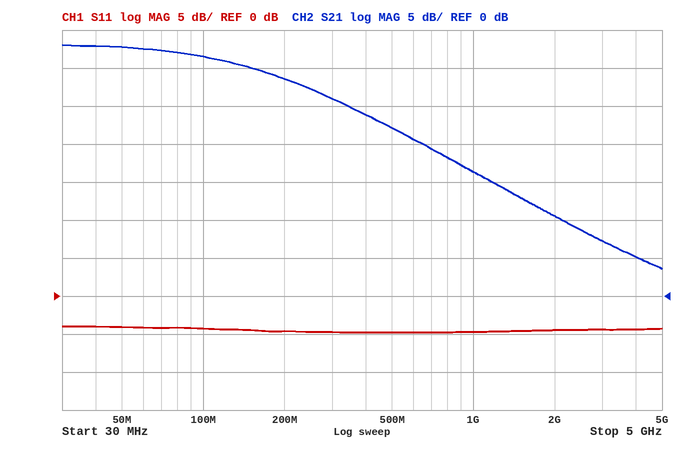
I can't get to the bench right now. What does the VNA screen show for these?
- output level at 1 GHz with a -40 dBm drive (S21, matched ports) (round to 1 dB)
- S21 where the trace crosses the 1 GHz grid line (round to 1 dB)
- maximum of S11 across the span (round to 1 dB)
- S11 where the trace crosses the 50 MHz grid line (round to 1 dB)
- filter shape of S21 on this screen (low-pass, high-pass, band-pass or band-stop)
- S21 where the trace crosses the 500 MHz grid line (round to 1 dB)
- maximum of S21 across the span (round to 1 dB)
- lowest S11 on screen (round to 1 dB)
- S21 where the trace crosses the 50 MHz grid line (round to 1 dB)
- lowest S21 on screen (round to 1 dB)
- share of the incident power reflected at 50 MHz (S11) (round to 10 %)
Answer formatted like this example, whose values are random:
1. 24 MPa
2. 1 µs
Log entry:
1. -24 dBm
2. 16 dB
3. -4 dB
4. -4 dB
5. low-pass
6. 22 dB
7. 33 dB
8. -5 dB
9. 33 dB
10. 4 dB
11. 40 %
